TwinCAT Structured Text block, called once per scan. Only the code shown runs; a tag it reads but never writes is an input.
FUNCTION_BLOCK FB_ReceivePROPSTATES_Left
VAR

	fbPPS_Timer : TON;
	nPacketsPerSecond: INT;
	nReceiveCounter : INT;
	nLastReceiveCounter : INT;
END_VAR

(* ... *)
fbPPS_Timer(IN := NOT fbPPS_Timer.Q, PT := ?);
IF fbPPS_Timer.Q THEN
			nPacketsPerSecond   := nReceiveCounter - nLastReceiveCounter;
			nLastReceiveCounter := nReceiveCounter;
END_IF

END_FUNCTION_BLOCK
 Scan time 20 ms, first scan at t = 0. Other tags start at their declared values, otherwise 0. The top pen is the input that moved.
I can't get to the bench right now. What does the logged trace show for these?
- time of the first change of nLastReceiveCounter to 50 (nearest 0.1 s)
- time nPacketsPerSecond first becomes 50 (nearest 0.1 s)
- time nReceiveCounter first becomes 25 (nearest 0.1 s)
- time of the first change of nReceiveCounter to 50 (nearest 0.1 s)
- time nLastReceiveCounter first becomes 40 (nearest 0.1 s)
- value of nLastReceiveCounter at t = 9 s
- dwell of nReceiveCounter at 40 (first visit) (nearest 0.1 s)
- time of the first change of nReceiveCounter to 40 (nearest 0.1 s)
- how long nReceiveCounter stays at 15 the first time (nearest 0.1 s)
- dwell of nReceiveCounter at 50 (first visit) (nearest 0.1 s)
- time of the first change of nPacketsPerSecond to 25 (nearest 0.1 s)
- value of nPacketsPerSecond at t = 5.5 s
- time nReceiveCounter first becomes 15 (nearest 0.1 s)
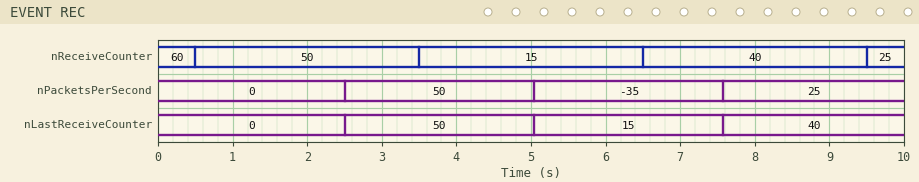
2.5 s
2.5 s
9.5 s
0.5 s
7.6 s
40
3.0 s
6.5 s
3.0 s
3.0 s
7.6 s
-35
3.5 s
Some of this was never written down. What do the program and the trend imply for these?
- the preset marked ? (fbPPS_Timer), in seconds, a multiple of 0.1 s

2.5 s
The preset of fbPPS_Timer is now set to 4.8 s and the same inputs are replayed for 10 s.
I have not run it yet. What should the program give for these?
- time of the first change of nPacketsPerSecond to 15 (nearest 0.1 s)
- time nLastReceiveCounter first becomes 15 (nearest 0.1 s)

4.8 s
4.8 s
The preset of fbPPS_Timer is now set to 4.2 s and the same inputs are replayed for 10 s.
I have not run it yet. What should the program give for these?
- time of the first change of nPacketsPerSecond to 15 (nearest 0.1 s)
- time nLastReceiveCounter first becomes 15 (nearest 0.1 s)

4.2 s
4.2 s
